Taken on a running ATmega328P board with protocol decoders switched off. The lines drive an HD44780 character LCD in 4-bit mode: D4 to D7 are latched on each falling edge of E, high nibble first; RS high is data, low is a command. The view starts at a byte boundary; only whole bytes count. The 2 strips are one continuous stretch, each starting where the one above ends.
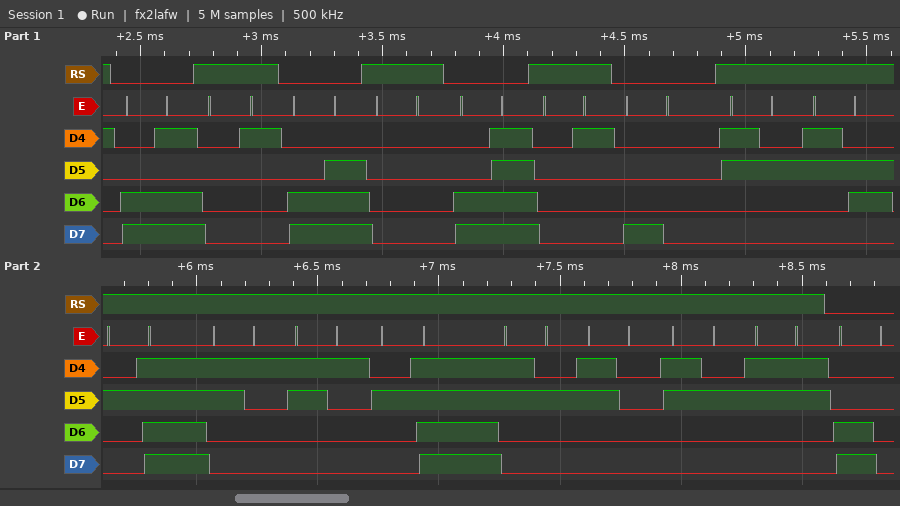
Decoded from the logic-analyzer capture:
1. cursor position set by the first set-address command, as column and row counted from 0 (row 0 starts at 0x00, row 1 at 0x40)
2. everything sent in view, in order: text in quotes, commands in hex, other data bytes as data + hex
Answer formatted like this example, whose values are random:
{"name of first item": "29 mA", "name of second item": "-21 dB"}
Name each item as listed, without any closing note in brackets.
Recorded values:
{"cursor position set by the first set-address command, as column and row counted from 0": "column 13, row 1", "everything sent in view, in order: text in quotes, commands in hex, other data bytes as data + hex": "0xCD data 01 0xCE data 00 0xCF data 01 0x80 \"26/11/2023\" 0xC0"}
